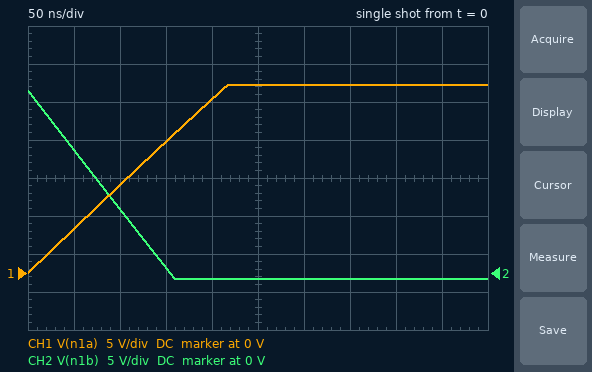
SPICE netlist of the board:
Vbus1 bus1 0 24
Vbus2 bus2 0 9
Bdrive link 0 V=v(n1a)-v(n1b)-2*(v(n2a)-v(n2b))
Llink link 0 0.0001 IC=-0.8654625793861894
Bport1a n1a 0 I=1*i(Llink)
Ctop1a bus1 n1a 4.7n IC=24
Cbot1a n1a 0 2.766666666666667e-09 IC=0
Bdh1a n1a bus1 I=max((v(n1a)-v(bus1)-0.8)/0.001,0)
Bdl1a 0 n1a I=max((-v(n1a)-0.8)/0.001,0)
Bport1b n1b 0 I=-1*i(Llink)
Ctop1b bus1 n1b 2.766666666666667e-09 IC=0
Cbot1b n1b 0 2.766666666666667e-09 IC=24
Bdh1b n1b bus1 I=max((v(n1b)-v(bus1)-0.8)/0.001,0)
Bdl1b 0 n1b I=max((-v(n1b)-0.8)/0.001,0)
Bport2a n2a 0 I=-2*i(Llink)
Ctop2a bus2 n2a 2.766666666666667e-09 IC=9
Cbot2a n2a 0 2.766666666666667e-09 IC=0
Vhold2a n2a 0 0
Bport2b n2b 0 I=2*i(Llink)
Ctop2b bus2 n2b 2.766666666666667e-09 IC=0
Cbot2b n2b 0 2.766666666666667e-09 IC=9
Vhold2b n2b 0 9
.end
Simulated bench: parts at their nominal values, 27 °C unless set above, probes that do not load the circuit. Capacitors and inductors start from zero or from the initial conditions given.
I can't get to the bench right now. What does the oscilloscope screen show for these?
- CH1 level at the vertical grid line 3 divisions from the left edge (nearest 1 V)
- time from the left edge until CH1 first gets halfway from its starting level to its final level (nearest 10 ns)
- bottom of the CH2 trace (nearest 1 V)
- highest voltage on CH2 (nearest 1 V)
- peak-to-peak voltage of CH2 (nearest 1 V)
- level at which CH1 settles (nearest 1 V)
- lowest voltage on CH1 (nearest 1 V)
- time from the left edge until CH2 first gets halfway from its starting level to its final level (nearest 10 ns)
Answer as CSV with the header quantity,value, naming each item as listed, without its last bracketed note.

quantity,value
CH1 level at the vertical grid line 3 divisions from the left edge,17 V
time from the left edge until CH1 first gets halfway from its starting level to its final level,110 ns
bottom of the CH2 trace,-1 V
highest voltage on CH2,24 V
peak-to-peak voltage of CH2,25 V
level at which CH1 settles,25 V
lowest voltage on CH1,0 V
time from the left edge until CH2 first gets halfway from its starting level to its final level,80 ns
